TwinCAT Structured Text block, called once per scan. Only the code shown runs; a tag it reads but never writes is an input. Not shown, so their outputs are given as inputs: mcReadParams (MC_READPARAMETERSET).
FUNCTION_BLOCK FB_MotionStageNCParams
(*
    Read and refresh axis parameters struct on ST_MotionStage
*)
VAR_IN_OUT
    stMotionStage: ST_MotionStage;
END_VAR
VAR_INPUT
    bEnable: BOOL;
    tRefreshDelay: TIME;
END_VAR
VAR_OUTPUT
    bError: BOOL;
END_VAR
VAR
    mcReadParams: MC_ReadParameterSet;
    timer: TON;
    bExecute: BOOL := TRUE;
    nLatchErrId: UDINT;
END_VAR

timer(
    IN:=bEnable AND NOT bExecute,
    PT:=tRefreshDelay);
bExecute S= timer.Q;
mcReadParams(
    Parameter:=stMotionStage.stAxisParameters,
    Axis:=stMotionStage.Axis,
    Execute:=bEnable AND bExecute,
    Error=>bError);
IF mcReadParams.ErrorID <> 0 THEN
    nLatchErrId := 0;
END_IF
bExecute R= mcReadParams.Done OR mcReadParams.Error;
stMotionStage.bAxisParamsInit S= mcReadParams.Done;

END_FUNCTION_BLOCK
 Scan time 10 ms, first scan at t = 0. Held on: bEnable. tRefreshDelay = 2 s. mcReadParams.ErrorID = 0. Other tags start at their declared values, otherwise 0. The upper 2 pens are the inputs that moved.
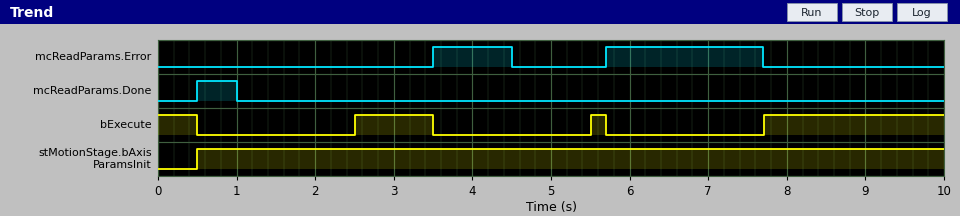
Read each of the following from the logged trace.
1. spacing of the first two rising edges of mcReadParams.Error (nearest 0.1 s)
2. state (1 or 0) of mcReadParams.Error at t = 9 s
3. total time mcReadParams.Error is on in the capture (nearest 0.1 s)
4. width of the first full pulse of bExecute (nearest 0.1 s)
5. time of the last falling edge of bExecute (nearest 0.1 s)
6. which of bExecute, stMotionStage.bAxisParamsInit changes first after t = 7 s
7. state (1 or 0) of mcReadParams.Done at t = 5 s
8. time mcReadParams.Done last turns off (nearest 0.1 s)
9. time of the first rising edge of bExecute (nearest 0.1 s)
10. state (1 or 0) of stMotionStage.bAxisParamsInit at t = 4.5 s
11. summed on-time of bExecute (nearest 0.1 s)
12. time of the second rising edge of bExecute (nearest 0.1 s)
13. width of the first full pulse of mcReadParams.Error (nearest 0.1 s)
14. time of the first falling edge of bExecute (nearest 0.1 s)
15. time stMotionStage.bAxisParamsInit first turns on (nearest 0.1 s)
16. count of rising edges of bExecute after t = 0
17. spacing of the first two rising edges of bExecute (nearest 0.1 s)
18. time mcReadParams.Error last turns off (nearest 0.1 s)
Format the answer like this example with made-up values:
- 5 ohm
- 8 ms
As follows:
- 2.2 s
- 0
- 3.0 s
- 1.0 s
- 5.7 s
- bExecute
- 0
- 1.0 s
- 2.5 s
- 1
- 4.0 s
- 5.5 s
- 1.0 s
- 0.5 s
- 0.5 s
- 3
- 3.0 s
- 7.7 s
